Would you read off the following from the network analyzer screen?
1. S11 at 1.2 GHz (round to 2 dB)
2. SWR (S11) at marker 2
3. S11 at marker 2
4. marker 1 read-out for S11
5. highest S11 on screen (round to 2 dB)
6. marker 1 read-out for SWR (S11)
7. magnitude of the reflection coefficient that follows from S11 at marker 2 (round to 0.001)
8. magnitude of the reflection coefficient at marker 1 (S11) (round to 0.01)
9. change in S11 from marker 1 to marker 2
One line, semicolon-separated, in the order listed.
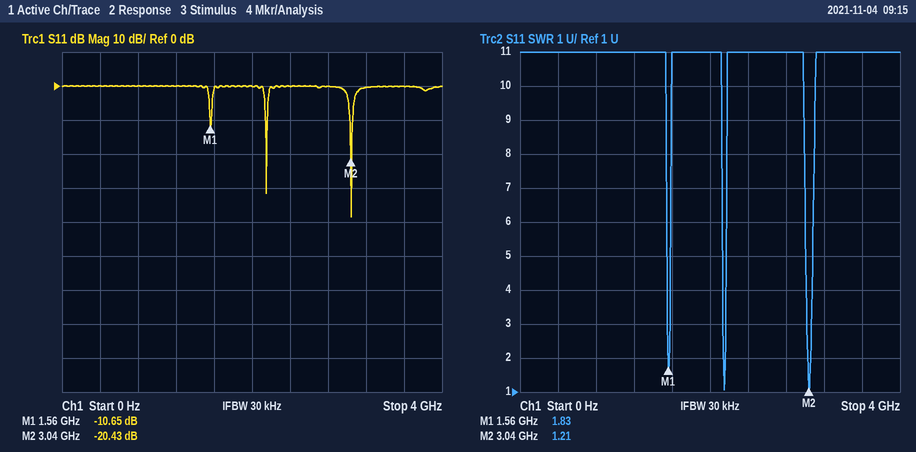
0 dB; 1.21; -20.43 dB; -10.65 dB; 0 dB; 1.83; 0.095; 0.29; -9.78 dB
